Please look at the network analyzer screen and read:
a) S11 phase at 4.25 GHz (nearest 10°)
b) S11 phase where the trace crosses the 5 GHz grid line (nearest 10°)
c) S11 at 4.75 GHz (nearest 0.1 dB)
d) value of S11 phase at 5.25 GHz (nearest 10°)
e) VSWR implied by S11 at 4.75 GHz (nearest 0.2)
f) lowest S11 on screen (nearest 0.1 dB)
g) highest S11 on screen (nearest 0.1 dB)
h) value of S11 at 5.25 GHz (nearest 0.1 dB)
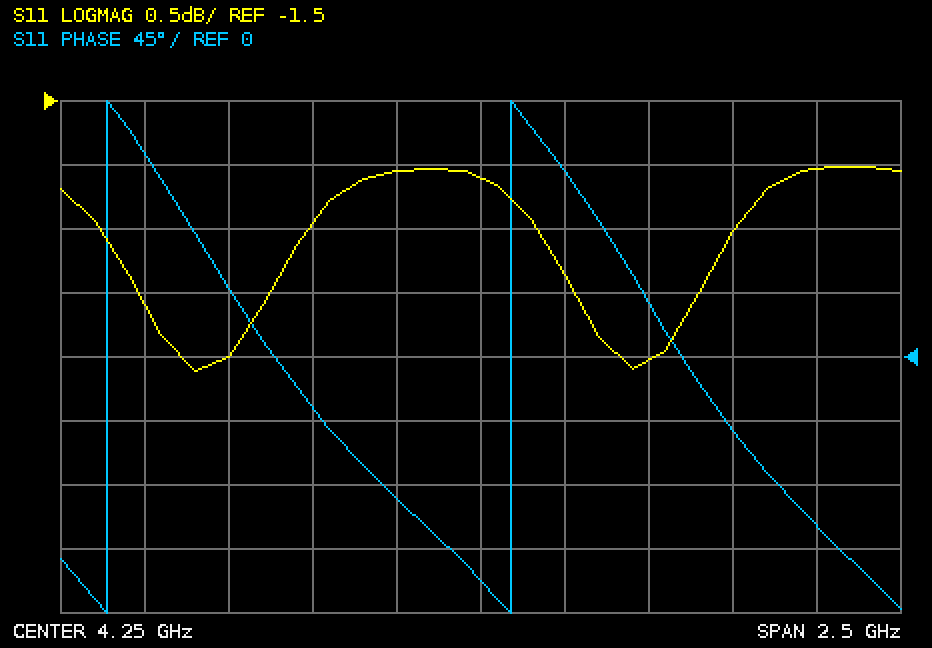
-160°
-50°
-3.5 dB
-120°
5.0
-3.6 dB
-2.0 dB
-2.0 dB
